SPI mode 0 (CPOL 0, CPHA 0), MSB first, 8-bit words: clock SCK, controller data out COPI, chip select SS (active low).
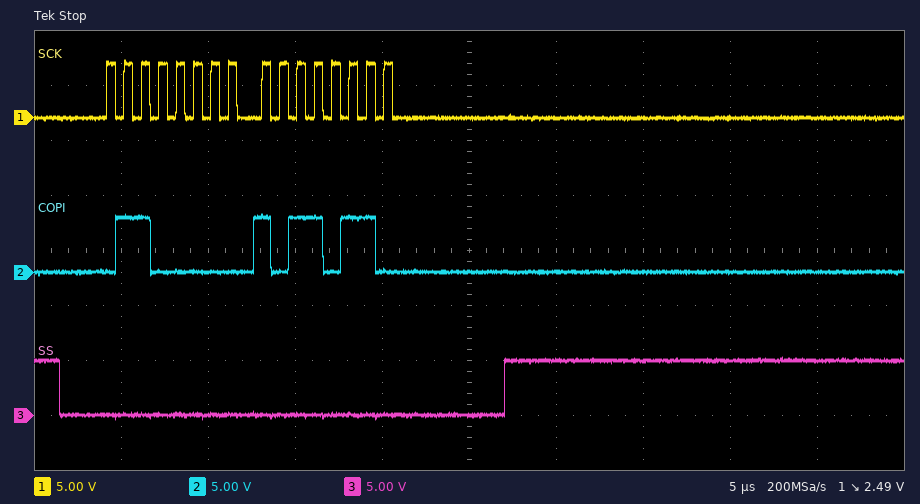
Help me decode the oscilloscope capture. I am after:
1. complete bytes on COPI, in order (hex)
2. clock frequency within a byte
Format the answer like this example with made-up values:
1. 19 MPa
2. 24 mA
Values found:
1. 60 B6
2. 1 MHz
